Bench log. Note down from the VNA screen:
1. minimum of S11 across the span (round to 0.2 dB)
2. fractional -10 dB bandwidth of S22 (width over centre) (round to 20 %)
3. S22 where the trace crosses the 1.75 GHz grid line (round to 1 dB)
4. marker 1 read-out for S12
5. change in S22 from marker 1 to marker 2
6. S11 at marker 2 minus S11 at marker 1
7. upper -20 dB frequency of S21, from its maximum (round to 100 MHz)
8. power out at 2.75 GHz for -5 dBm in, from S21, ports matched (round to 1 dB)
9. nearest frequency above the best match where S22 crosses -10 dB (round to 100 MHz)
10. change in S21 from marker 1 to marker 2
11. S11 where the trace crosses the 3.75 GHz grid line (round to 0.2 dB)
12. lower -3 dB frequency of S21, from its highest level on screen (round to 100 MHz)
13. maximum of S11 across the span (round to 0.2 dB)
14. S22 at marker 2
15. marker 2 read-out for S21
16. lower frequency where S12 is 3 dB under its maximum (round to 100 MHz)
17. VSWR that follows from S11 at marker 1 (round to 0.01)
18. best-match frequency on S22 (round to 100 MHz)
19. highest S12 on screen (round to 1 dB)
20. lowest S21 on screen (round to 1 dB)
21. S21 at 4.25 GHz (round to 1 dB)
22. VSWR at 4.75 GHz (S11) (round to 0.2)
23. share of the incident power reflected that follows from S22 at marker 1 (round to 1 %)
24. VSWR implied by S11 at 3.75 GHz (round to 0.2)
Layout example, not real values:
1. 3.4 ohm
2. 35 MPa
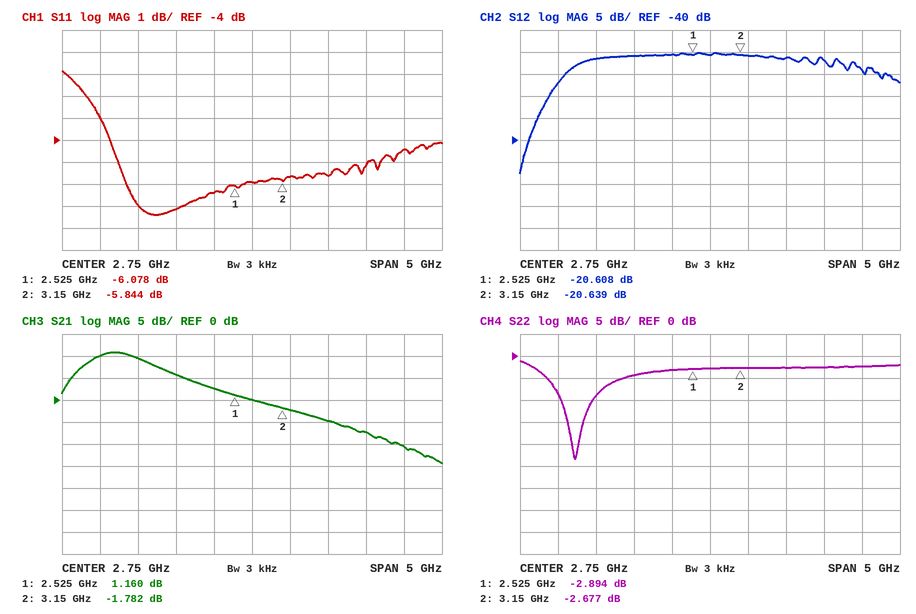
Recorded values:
1. -7.4 dB
2. 40 %
3. -4 dB
4. -20.608 dB
5. 0.217 dB
6. 0.234 dB
7. 4.5 GHz
8. -5 dBm
9. 1.2 GHz
10. -2.942 dB
11. -5.6 dB
12. 500 MHz
13. -0.8 dB
14. -2.677 dB
15. -1.782 dB
16. 1.0 GHz
17. 2.97
18. 1.0 GHz
19. -20 dB
20. -14 dB
21. -7 dB
22. 4.0
23. 51 %
24. 3.2
